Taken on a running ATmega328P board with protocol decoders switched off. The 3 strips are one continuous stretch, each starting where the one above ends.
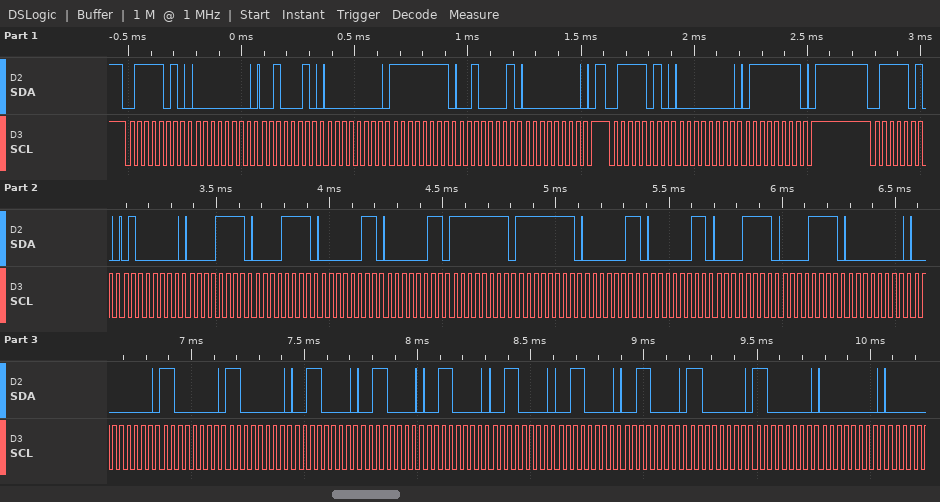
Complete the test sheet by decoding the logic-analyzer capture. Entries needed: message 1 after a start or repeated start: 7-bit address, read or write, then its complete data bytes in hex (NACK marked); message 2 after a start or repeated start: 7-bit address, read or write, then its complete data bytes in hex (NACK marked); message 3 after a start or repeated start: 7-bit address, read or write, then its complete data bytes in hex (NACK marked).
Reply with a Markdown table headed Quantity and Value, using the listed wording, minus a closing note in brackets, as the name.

| Quantity | Value |
|---|---|
| message 1 after a start or repeated start: 7-bit address, read or write, then its complete data bytes in hex | 0x3D write: 00 22 00 FF 21 00 |
| message 2 after a start or repeated start: 7-bit address, read or write, then its complete data bytes in hex | 0x3D write: 00 7F |
| message 3 after a start or repeated start: 7-bit address, read or write, then its complete data bytes in hex | 0x3D write: 40 0F 0F 03 03 FF FF 03 03 0F 0F 00 00 C0 C0 30 30 30 30 30 30 C0 C0 00 |
